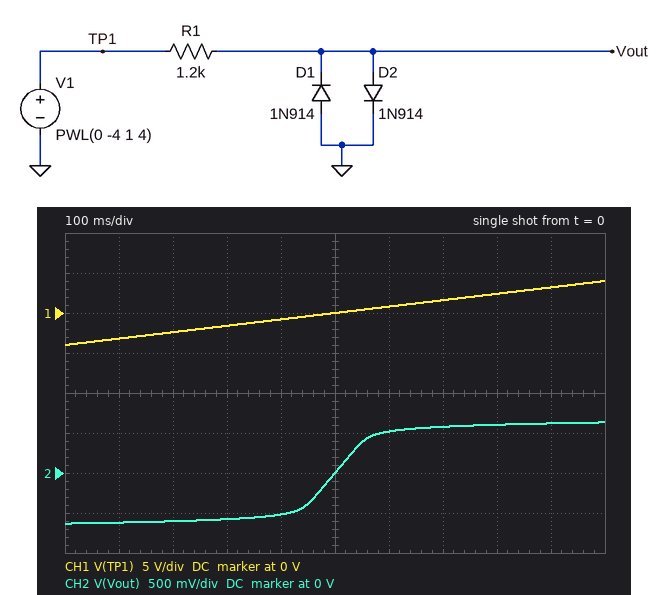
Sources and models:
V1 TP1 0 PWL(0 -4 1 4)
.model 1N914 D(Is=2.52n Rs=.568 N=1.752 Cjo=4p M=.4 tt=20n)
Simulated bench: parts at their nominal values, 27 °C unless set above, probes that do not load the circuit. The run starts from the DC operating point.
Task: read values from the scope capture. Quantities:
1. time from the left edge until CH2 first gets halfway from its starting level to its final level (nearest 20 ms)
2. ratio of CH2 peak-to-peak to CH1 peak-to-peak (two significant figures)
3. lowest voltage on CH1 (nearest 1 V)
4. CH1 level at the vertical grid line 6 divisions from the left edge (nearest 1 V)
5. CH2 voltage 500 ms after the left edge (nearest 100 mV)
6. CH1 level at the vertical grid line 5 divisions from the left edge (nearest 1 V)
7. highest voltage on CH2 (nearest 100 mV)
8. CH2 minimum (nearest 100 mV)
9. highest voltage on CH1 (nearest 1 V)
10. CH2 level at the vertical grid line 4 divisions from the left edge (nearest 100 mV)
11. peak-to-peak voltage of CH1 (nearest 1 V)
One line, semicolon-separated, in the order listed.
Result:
500 ms; 0.16; -4 V; 1 V; 0 V; 0 V; 600 mV; -600 mV; 4 V; -500 mV; 8 V
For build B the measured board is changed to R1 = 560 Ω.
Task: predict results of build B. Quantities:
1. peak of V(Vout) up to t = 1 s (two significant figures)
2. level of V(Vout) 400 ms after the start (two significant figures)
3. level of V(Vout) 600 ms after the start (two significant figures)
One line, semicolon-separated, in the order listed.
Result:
670 mV; -550 mV; 550 mV
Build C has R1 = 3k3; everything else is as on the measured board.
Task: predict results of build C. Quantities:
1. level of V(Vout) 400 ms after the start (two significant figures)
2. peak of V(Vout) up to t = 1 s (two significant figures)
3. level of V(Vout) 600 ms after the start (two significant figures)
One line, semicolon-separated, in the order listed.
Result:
-480 mV; 590 mV; 480 mV
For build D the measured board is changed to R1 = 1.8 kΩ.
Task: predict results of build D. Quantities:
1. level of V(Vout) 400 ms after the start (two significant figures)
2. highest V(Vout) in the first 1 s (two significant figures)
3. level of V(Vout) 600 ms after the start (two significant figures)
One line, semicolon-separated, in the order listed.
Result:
-500 mV; 610 mV; 500 mV
